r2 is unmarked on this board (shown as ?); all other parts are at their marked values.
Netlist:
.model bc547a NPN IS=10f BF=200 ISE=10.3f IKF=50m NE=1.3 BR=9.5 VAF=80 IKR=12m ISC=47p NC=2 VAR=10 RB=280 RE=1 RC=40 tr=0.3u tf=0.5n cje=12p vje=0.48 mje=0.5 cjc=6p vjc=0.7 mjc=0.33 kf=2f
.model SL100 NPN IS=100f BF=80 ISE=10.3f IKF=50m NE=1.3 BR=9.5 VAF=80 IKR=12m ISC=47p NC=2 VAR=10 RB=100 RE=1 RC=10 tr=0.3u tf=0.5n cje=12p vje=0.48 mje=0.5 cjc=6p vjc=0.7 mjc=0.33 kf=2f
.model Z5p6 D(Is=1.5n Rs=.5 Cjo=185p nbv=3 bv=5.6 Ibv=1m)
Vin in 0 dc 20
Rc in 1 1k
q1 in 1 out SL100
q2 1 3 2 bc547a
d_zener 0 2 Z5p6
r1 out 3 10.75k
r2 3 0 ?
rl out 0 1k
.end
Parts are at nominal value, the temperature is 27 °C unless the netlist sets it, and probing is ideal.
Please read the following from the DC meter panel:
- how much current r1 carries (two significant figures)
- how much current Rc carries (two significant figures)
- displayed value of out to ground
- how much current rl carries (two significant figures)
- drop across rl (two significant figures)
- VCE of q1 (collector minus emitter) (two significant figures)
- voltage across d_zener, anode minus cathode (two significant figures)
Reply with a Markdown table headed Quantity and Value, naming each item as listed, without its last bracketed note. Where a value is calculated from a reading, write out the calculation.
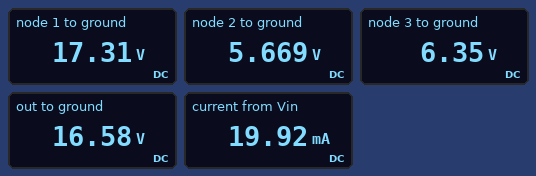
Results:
| Quantity | Value |
|---|---|
| how much current r1 carries | (16.58 V - 6.35 V) / 10.75 kΩ = 950 µA |
| how much current Rc carries | (20 V - 17.31 V) / 1 kΩ = 2.7 mA |
| displayed value of out to ground | 16.58 V |
| how much current rl carries | (16.58 V) / 1 kΩ = 17 mA |
| drop across rl | 16.58 V = 17 V |
| VCE of q1 (collector minus emitter) | 20 V - 16.58 V = 3.4 V |
| voltage across d_zener, anode minus cathode | 0 V - 5.669 V = -5.7 V |
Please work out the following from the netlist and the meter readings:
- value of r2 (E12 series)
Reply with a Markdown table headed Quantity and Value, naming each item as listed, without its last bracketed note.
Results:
| Quantity | Value |
|---|---|
| value of r2 | 6.8 kΩ |
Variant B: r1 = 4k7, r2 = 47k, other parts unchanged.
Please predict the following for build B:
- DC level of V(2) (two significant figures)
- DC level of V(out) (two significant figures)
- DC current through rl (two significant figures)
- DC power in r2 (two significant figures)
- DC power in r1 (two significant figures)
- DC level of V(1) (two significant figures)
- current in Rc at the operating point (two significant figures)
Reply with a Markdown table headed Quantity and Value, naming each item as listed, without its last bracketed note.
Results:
| Quantity | Value |
|---|---|
| DC level of V(2) | 5.8 V |
| DC level of V(out) | 7.7 V |
| DC current through rl | 7.7 mA |
| DC power in r2 | 920 µW |
| DC power in r1 | 270 µW |
| DC level of V(1) | 8.4 V |
| current in Rc at the operating point | 12 mA |
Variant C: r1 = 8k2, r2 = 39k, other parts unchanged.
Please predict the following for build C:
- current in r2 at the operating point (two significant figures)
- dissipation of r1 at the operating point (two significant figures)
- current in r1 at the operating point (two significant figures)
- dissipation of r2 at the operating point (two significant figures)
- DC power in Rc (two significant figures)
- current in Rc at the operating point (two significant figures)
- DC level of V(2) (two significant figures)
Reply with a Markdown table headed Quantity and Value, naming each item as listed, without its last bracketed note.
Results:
| Quantity | Value |
|---|---|
| current in r2 at the operating point | 170 µA |
| dissipation of r1 at the operating point | 540 µW |
| current in r1 at the operating point | 260 µA |
| dissipation of r2 at the operating point | 1.1 mW |
| DC power in Rc | 110 mW |
| current in Rc at the operating point | 11 mA |
| DC level of V(2) | 5.8 V |
